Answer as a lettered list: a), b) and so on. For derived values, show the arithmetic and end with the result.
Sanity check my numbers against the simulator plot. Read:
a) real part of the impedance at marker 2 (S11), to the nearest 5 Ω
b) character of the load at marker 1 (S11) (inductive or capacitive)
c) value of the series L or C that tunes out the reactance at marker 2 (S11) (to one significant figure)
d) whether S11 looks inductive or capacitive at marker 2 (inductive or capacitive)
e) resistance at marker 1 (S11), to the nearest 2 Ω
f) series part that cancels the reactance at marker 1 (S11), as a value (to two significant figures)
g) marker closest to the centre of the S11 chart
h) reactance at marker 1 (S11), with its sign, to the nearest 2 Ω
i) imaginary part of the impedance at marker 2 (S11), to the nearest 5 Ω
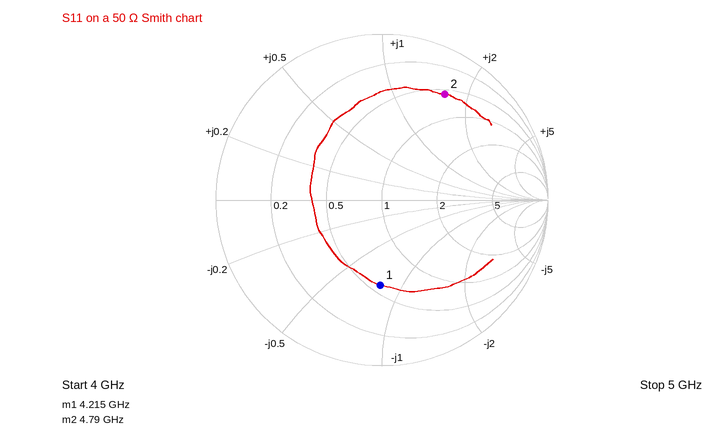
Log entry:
a) 30 Ω
b) capacitive
c) C = 1/(2π × 4.79 GHz × 80 Ω) ≈ 415 fF, so 400 fF to one significant figure
d) inductive
e) 28 Ω
f) L = 40 Ω/(2π × 4.215 GHz) ≈ 1.5 nH
g) marker 1
h) -40 Ω
i) +80 Ω
